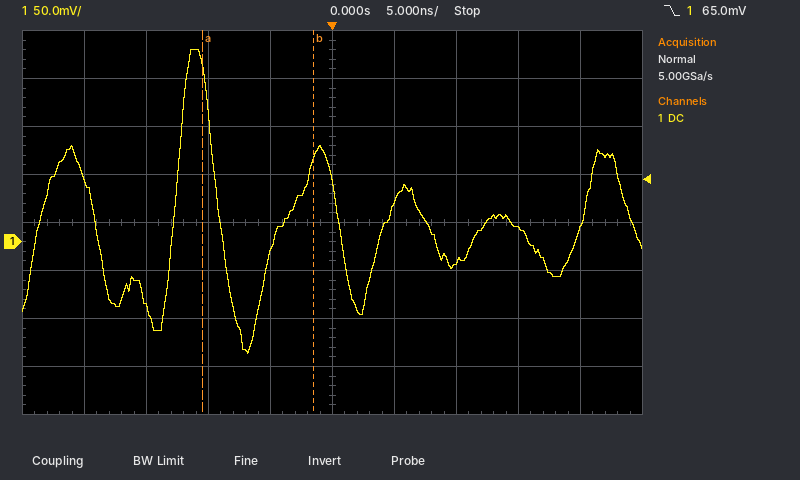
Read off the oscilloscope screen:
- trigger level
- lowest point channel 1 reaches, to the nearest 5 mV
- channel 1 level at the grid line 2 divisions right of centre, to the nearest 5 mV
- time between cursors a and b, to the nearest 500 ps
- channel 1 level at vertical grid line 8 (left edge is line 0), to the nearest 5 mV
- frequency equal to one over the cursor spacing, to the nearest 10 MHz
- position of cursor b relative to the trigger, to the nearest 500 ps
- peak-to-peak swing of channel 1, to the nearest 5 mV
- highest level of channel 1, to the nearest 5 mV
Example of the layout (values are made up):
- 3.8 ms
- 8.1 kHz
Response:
- 65.0 mV
- -115 mV
- -20 mV
- 9.0 ns
- 15 mV
- 110 MHz
- -1.5 ns
- 315 mV
- 200 mV
